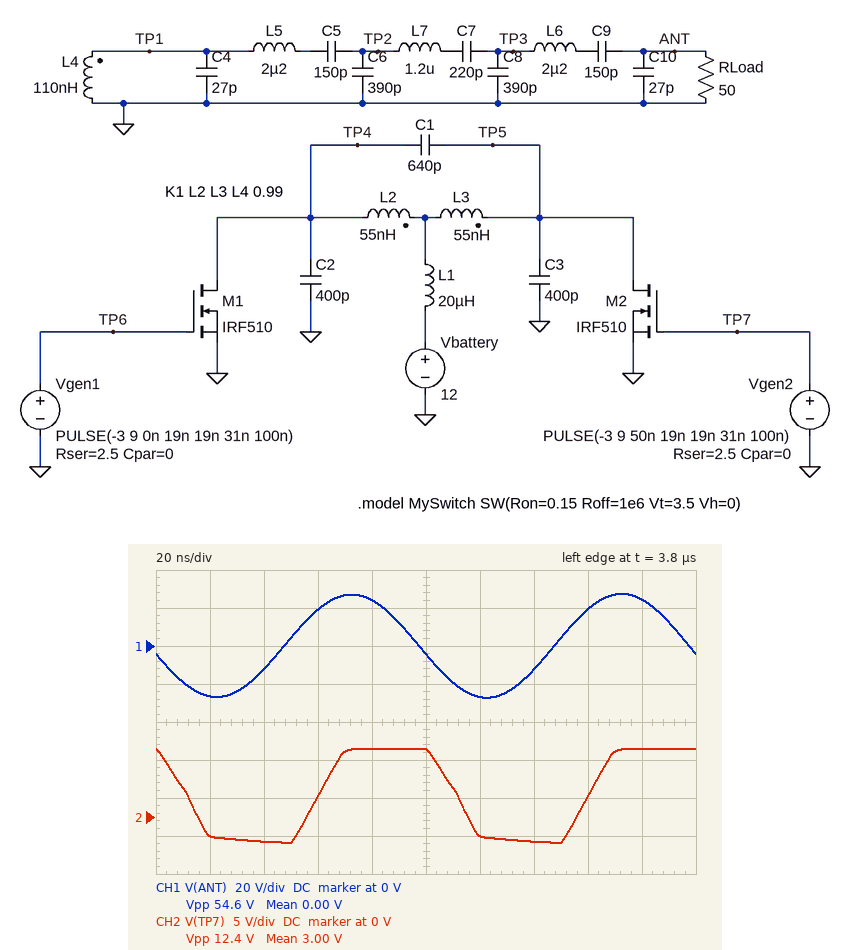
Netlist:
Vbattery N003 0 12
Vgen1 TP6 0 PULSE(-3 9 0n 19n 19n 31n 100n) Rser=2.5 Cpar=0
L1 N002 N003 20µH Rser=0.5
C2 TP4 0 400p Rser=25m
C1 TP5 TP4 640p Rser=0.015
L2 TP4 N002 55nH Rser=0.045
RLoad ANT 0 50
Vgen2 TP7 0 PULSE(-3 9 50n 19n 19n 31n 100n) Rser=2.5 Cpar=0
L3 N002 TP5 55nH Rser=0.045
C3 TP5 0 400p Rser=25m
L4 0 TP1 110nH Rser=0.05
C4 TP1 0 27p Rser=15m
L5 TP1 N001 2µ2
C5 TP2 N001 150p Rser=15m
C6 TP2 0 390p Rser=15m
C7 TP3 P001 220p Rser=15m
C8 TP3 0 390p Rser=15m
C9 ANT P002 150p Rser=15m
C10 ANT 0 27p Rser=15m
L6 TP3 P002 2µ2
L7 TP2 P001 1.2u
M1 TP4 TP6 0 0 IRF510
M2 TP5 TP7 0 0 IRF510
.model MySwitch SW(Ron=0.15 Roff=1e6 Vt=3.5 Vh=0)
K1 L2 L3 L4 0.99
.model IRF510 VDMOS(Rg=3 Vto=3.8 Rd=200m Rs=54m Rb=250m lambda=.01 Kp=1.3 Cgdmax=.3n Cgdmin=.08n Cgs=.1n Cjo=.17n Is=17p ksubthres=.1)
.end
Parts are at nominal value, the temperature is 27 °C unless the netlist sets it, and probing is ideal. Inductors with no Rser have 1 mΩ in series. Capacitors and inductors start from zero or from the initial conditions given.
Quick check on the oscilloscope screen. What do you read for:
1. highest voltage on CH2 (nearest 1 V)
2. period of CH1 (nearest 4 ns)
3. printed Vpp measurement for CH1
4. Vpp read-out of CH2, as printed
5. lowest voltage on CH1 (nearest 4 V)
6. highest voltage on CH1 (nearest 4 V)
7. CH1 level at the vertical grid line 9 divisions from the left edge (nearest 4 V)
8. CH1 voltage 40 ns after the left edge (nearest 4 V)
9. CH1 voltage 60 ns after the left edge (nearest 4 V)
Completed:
9 V
100 ns
54.6 V
12.4 V
-28 V
28 V
24 V
-12 V
20 V
